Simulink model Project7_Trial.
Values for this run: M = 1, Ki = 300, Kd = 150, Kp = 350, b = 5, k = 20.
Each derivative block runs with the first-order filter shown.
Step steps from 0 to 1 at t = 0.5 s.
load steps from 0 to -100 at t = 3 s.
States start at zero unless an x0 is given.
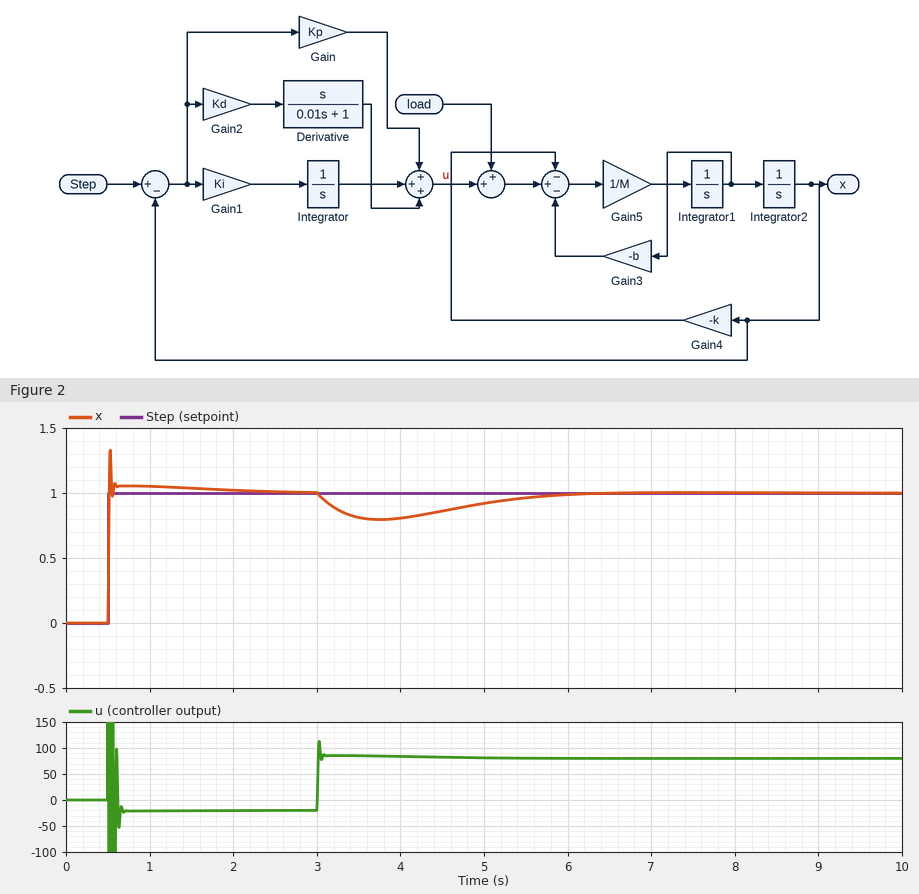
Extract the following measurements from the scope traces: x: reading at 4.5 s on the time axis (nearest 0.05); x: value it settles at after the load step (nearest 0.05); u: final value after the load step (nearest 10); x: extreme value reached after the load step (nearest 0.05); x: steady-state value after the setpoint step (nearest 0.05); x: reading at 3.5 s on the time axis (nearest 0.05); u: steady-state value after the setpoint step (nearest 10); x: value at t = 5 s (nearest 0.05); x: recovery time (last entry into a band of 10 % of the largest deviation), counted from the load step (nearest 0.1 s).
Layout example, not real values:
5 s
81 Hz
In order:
0.85
1.00
80
0.80
1.00
0.80
-20
0.90
2.8 s
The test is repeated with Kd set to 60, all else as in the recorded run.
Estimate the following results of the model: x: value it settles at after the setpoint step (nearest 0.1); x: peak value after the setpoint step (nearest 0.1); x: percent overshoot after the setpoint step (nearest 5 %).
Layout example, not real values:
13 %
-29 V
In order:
1.0
1.3
30 %
